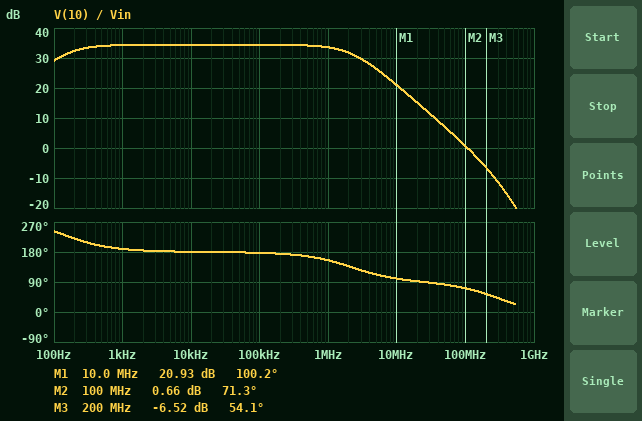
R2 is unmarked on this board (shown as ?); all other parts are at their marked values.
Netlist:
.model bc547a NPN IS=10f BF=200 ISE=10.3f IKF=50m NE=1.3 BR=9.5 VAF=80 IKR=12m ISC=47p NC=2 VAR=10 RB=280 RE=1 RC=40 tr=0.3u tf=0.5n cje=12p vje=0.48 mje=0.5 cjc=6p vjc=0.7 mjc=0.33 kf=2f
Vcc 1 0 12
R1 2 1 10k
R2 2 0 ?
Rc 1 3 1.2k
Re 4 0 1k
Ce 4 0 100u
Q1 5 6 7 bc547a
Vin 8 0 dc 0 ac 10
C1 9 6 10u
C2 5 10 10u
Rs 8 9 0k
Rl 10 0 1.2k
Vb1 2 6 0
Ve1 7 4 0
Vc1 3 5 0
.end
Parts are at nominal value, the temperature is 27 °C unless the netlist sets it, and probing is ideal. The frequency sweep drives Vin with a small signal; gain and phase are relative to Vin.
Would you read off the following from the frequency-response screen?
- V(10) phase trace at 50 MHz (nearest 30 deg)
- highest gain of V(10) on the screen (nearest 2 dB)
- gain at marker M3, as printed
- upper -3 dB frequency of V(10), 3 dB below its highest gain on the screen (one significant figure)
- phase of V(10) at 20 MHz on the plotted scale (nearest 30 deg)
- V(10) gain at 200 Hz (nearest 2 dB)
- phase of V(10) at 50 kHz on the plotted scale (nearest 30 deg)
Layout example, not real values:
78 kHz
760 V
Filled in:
90 deg
34 dB
-6.52 dB
2 MHz
90 deg
32 dB
180 deg
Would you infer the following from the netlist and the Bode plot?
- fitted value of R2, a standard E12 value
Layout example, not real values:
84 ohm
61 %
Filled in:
5.6 kΩ
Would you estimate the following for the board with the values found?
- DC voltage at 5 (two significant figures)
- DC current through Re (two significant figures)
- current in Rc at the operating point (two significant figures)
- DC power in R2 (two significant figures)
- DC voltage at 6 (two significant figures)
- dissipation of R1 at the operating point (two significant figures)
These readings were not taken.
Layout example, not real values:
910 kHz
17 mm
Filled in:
7.8 V
3.5 mA
3.5 mA
3.2 mW
4.2 V
6.1 mW
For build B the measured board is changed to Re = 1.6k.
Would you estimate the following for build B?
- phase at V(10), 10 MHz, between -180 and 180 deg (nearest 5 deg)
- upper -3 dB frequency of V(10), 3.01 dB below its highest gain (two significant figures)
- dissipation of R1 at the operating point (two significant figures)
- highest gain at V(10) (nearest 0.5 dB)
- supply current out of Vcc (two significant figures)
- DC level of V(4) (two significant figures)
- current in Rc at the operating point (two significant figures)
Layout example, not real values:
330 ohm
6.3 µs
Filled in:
105 deg
3.0 MHz
6.0 mW
31.5 dB
3.0 mA
3.6 V
2.2 mA
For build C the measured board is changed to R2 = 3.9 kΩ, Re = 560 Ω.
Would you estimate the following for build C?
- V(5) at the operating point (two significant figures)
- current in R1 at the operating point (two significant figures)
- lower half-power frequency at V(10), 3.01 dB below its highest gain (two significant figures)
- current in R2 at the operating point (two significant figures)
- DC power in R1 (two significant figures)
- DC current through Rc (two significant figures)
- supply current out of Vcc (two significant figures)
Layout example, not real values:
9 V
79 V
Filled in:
6.6 V
870 µA
180 Hz
840 µA
7.6 mW
4.5 mA
5.4 mA
